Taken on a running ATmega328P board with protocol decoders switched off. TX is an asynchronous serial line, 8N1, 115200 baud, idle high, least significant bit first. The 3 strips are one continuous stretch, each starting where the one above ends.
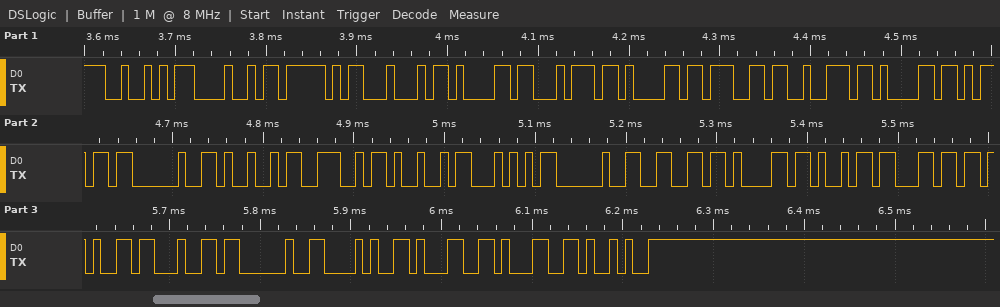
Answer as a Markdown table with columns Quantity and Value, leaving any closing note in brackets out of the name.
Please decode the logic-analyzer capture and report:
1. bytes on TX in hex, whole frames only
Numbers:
| Quantity | Value |
|---|---|
| bytes on TX in hex, whole frames only | 0x52 0x48 0x5F 0x44 0x61 0x74 0x61 0x67 0x72 0x61 0x6D 0x20 0x49 0x4E 0x49 0x54 0x20 0x66 0x61 0x69 0x6C 0x65 0x64 0x20 0x28 0x31 0x31 0x29 |
